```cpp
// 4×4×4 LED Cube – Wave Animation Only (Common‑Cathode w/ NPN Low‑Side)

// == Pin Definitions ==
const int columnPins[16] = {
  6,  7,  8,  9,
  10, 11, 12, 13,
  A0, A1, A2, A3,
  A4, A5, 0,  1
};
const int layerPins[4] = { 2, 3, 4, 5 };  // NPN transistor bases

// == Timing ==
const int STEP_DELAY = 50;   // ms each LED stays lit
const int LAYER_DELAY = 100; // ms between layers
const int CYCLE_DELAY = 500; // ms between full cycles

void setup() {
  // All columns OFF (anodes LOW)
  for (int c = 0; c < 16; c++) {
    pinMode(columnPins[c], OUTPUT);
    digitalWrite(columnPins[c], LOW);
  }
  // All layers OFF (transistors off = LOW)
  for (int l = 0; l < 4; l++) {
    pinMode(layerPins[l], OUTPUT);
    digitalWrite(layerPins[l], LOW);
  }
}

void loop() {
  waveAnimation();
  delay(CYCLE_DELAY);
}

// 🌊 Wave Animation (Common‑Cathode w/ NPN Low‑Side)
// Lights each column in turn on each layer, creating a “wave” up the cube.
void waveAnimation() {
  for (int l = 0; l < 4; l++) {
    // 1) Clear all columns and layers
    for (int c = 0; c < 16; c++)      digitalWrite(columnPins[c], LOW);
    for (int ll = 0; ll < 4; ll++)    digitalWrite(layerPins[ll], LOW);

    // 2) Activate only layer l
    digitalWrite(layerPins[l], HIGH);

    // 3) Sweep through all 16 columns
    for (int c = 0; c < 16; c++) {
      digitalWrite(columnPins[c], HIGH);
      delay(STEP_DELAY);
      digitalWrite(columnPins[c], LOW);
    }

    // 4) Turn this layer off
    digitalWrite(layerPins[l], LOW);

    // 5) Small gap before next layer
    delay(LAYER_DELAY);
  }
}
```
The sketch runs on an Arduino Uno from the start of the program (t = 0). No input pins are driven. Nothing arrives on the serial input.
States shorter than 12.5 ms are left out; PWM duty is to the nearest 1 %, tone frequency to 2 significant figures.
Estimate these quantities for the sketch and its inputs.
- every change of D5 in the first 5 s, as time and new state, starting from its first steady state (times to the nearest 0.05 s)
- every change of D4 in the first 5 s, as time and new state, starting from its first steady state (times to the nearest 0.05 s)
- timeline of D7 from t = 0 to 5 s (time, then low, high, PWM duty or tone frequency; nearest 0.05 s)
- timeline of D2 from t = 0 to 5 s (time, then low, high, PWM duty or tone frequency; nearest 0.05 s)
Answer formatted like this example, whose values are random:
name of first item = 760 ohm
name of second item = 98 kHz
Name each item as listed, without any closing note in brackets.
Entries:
every change of D5 in the first 5 s, as time and new state, starting from its first steady state = 0 s low; 2.7 s high; 3.5 s low
every change of D4 in the first 5 s, as time and new state, starting from its first steady state = 0 s low; 1.8 s high; 2.6 s low
timeline of D7 from t = 0 to 5 s = 0 s low; 0.05 s high; 0.1 s low; 0.95 s high; 1 s low; 1.85 s high; 1.9 s low; 2.75 s high; 2.8 s low; 4.15 s high; 4.2 s low
timeline of D2 from t = 0 to 5 s = 0 s high; 0.8 s low; 4.1 s high; 4.9 s low
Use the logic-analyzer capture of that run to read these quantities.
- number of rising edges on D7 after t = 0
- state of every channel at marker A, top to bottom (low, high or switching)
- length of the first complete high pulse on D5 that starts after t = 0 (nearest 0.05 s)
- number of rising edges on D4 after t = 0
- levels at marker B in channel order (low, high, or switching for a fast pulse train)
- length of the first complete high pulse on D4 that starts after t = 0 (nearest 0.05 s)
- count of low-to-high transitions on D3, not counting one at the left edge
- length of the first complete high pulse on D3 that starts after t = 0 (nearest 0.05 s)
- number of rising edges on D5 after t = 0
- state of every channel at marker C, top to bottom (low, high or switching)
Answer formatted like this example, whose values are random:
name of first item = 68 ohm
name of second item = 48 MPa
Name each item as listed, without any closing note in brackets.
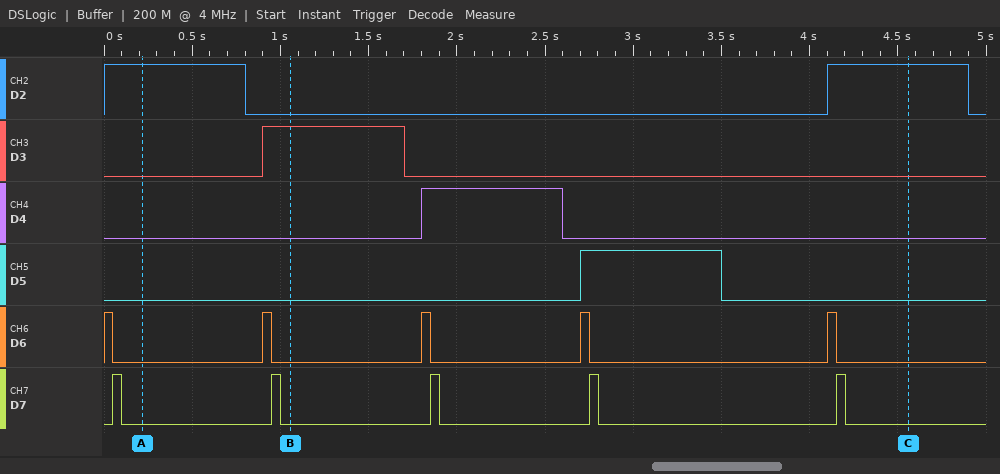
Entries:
number of rising edges on D7 after t = 0 = 5
state of every channel at marker A, top to bottom = D2 high, D3 low, D4 low, D5 low, D6 low, D7 low
length of the first complete high pulse on D5 that starts after t = 0 = 0.80 s
number of rising edges on D4 after t = 0 = 1
levels at marker B in channel order = D2 low, D3 high, D4 low, D5 low, D6 low, D7 low
length of the first complete high pulse on D4 that starts after t = 0 = 0.80 s
count of low-to-high transitions on D3, not counting one at the left edge = 1
length of the first complete high pulse on D3 that starts after t = 0 = 0.80 s
number of rising edges on D5 after t = 0 = 1
state of every channel at marker C, top to bottom = D2 high, D3 low, D4 low, D5 low, D6 low, D7 low
